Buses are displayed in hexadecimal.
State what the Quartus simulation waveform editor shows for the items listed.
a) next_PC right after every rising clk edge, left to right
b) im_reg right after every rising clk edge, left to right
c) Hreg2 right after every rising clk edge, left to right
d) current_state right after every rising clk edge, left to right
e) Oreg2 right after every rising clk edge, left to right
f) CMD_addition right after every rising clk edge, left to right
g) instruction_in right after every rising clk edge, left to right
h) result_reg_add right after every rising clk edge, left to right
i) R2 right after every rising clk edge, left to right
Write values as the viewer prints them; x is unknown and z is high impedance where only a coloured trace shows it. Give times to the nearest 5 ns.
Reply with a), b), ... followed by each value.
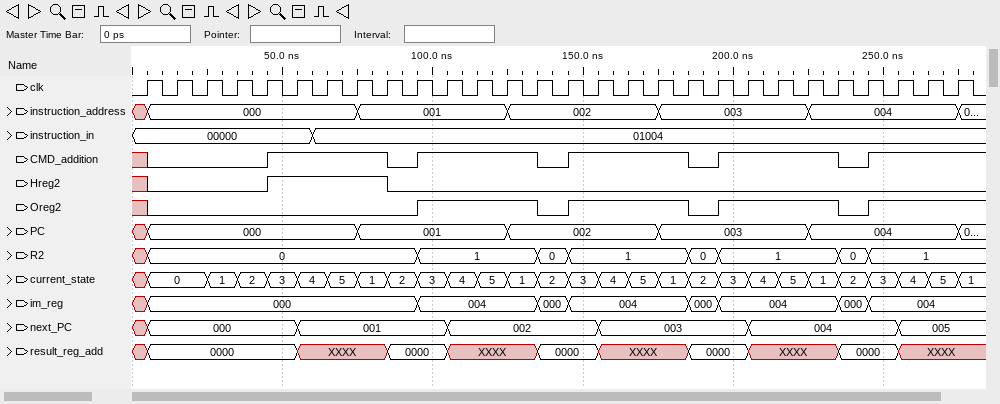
a) 000, 000, 000, 000, 000, 001, 001, 001, 001, 001, 002, 002, 002, 002, 002, 003, 003, 003, 003, 003, 004, 004, 004, 004, 004, 005, 005, 005
b) 000, 000, 000, 000, 000, 000, 000, 000, 000, 004, 004, 004, 004, 000, 004, 004, 004, 004, 000, 004, 004, 004, 004, 000, 004, 004, 004, 004
c) 0 0 0 0 1 1 1 1 0 0 0 0 0 0 0 0 0 0 0 0 0 0 0 0 0 0 0 0
d) 0, 0, 1, 2, 3, 4, 5, 1, 2, 3, 4, 5, 1, 2, 3, 4, 5, 1, 2, 3, 4, 5, 1, 2, 3, 4, 5, 1
e) 0 0 0 0 0 0 0 0 0 1 1 1 1 0 1 1 1 1 0 1 1 1 1 0 1 1 1 1
f) 0 0 0 0 1 1 1 1 0 1 1 1 1 0 1 1 1 1 0 1 1 1 1 0 1 1 1 1
g) 00000, 00000, 00000, 00000, 00000, 00000, 01004, 01004, 01004, 01004, 01004, 01004, 01004, 01004, 01004, 01004, 01004, 01004, 01004, 01004, 01004, 01004, 01004, 01004, 01004, 01004, 01004, 01004
h) 0000, 0000, 0000, 0000, 0000, XXXX, XXXX, XXXX, 0000, 0000, XXXX, XXXX, XXXX, 0000, 0000, XXXX, XXXX, XXXX, 0000, 0000, XXXX, XXXX, XXXX, 0000, 0000, XXXX, XXXX, XXXX
i) 0, 0, 0, 0, 0, 0, 0, 0, 0, 1, 1, 1, 1, 0, 1, 1, 1, 1, 0, 1, 1, 1, 1, 0, 1, 1, 1, 1
